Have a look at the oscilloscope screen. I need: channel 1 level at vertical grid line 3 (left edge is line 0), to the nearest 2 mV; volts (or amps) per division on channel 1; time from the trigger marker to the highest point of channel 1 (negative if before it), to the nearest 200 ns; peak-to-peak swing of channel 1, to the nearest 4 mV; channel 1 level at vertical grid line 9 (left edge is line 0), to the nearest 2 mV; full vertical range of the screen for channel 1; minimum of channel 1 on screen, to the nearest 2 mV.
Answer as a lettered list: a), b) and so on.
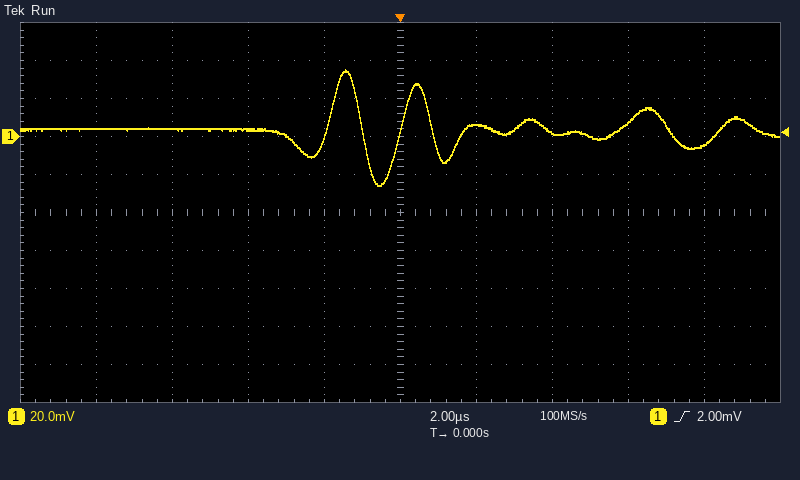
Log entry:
a) 4 mV
b) 20 mV
c) -1.4 µs
d) 60 mV
e) -4 mV
f) 200 mV
g) -26 mV
